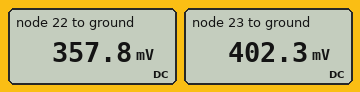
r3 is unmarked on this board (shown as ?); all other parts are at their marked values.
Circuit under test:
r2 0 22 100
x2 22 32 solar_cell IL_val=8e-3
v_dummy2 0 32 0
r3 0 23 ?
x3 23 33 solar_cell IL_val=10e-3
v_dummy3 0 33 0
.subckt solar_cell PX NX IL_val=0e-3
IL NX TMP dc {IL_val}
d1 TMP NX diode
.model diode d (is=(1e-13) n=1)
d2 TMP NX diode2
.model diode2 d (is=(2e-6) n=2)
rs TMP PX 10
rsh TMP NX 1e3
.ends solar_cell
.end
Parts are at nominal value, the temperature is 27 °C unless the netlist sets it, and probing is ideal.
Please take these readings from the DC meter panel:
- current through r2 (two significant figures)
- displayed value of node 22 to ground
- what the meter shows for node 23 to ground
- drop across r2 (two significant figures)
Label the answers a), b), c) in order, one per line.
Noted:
a) 3.6 mA
b) 357.8 mV
c) 402.3 mV
d) 360 mV
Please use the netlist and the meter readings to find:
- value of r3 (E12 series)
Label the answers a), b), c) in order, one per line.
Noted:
a) 180 Ω
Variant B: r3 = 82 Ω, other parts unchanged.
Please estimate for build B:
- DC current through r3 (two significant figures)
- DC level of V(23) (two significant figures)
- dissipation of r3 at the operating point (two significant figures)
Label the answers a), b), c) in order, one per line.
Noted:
a) 4.4 mA
b) 360 mV
c) 1.6 mW
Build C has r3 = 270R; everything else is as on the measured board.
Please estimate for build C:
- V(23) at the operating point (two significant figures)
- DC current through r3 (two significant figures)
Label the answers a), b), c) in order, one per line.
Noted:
a) 410 mV
b) 1.5 mA
